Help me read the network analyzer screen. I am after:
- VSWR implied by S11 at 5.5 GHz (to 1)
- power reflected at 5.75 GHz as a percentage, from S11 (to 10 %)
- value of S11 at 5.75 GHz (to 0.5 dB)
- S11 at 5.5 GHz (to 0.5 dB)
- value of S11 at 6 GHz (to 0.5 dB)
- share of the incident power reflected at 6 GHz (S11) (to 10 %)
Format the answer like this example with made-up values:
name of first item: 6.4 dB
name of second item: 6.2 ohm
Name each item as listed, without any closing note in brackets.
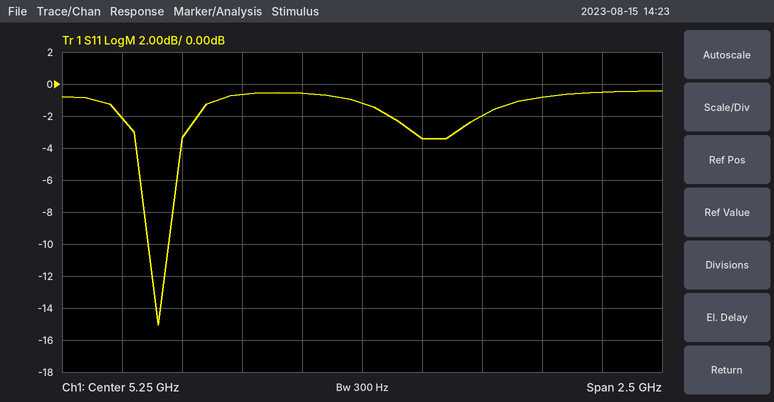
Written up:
VSWR implied by S11 at 5.5 GHz: 5
power reflected at 5.75 GHz as a percentage, from S11: 60 %
value of S11 at 5.75 GHz: -2.0 dB
S11 at 5.5 GHz: -3.5 dB
value of S11 at 6 GHz: -1.0 dB
share of the incident power reflected at 6 GHz (S11): 80 %
